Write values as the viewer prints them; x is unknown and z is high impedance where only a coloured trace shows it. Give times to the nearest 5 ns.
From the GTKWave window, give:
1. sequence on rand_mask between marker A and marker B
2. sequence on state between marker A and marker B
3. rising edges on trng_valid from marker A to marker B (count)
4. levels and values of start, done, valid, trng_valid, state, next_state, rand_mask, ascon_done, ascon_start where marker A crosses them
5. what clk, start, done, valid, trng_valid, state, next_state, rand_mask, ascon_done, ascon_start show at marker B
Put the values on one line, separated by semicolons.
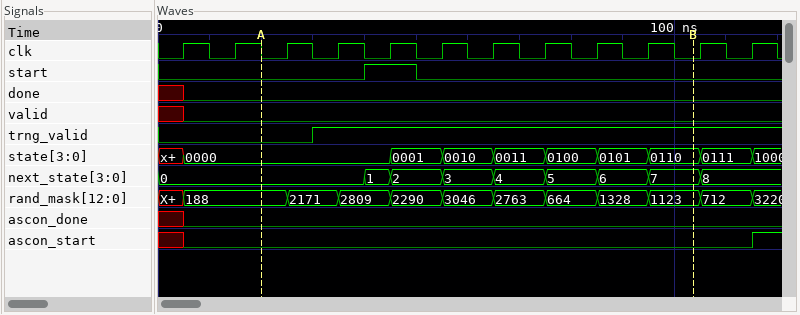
188, 2171, 2809, 2290, 3046, 2763, 664, 1328, 1123; 0000, 0001, 0010, 0011, 0100, 0101, 0110; 1; start=0, done=0, valid=0, trng_valid=0, state=0000, next_state=0, rand_mask=188, ascon_done=0, ascon_start=0; clk=0, start=0, done=0, valid=0, trng_valid=1, state=0110, next_state=7, rand_mask=1123, ascon_done=0, ascon_start=0
